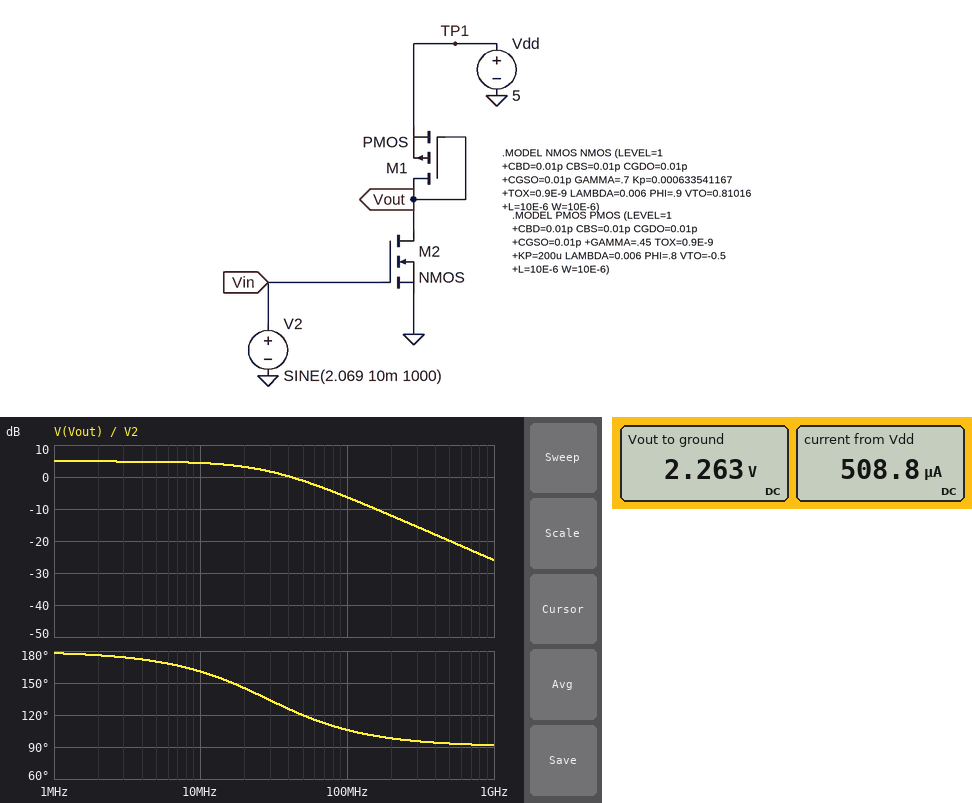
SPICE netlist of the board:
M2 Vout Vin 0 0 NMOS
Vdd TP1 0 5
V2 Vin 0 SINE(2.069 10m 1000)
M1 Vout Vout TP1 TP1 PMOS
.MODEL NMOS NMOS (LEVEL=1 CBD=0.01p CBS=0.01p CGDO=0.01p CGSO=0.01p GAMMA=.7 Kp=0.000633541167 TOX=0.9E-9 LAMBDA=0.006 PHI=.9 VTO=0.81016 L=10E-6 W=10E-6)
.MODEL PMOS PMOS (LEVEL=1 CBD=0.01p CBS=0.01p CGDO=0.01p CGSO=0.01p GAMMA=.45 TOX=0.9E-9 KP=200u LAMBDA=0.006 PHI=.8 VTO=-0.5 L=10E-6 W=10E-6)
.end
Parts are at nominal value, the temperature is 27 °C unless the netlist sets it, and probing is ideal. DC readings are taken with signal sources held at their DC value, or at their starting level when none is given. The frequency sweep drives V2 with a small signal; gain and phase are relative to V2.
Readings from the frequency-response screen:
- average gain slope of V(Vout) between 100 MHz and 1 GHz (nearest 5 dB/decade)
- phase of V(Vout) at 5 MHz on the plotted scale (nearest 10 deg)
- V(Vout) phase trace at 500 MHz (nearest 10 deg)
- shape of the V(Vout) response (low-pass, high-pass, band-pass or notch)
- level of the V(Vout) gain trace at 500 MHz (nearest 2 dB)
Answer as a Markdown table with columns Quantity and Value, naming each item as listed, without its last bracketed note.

| Quantity | Value |
|---|---|
| average gain slope of V(Vout) between 100 MHz and 1 GHz | -20 dB/decade |
| phase of V(Vout) at 5 MHz on the plotted scale | 170 deg |
| V(Vout) phase trace at 500 MHz | 90 deg |
| shape of the V(Vout) response | low-pass |
| level of the V(Vout) gain trace at 500 MHz | -20 dB |
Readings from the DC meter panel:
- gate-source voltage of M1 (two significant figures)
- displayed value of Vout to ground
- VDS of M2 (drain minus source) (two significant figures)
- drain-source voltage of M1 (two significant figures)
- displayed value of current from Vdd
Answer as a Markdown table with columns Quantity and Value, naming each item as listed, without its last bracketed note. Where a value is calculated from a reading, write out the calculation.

| Quantity | Value |
|---|---|
| gate-source voltage of M1 | 2.263 V - 5 V = -2.7 V |
| displayed value of Vout to ground | 2.263 V |
| VDS of M2 (drain minus source) | 2.263 V = 2.3 V |
| drain-source voltage of M1 | 2.263 V - 5 V = -2.7 V |
| displayed value of current from Vdd | 508.8 µA |
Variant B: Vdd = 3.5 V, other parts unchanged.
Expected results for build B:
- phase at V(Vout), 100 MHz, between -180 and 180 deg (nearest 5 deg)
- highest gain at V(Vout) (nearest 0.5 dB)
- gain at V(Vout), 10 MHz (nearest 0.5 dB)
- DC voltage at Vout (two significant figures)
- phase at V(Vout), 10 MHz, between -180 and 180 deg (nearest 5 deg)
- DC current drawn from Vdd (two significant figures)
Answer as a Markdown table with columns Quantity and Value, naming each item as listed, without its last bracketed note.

| Quantity | Value |
|---|---|
| phase at V(Vout), 100 MHz, between -180 and 180 deg | 55 deg |
| highest gain at V(Vout) | -1.5 dB |
| gain at V(Vout), 10 MHz | -2.0 dB |
| DC voltage at Vout | 880 mV |
| phase at V(Vout), 10 MHz, between -180 and 180 deg | 155 deg |
| DC current drawn from Vdd | 460 µA |
